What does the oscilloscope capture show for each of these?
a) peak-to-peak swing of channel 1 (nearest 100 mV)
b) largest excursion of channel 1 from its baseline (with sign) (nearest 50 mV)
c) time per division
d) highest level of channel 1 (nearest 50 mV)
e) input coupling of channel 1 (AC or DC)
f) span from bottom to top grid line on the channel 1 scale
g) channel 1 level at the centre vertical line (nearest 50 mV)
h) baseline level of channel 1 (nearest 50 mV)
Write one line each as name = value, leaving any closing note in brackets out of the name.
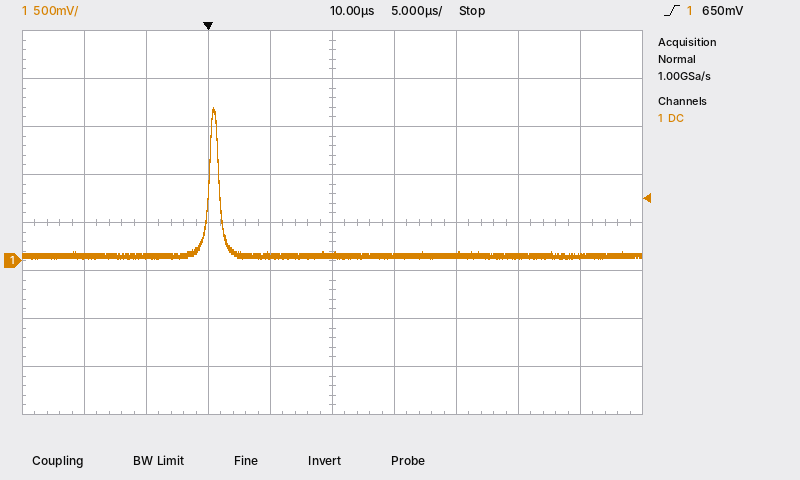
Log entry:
peak-to-peak swing of channel 1 = 1.60 V
largest excursion of channel 1 from its baseline (with sign) = +1.55 V
time per division = 5 µs
highest level of channel 1 = 1.60 V
input coupling of channel 1 = DC
span from bottom to top grid line on the channel 1 scale = 4 V
channel 1 level at the centre vertical line = 50 mV
baseline level of channel 1 = 50 mV
